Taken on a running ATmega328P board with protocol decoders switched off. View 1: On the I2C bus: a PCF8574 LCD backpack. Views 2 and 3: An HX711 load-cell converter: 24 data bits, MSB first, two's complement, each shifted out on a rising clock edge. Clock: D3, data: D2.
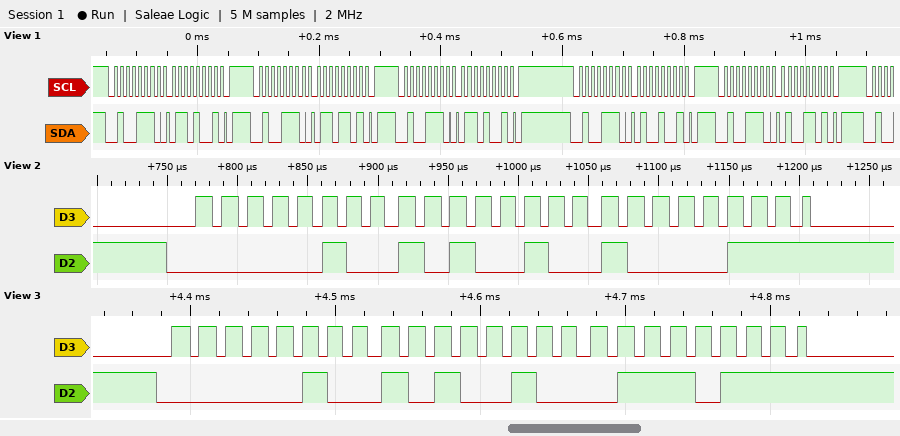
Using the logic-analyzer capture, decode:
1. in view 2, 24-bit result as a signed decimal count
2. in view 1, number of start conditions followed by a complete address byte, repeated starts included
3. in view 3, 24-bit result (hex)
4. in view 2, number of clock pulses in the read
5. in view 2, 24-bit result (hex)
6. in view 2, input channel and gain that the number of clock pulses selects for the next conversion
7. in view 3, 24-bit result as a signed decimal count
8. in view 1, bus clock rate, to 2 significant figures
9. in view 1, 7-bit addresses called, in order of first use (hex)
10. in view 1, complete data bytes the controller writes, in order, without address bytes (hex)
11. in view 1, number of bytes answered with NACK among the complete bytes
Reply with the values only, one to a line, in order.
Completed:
304263
5
0x04A477
25
0x04A487
channel A, gain 128
304247
100 kHz
0x27
69 6D 69 49 4D
0
